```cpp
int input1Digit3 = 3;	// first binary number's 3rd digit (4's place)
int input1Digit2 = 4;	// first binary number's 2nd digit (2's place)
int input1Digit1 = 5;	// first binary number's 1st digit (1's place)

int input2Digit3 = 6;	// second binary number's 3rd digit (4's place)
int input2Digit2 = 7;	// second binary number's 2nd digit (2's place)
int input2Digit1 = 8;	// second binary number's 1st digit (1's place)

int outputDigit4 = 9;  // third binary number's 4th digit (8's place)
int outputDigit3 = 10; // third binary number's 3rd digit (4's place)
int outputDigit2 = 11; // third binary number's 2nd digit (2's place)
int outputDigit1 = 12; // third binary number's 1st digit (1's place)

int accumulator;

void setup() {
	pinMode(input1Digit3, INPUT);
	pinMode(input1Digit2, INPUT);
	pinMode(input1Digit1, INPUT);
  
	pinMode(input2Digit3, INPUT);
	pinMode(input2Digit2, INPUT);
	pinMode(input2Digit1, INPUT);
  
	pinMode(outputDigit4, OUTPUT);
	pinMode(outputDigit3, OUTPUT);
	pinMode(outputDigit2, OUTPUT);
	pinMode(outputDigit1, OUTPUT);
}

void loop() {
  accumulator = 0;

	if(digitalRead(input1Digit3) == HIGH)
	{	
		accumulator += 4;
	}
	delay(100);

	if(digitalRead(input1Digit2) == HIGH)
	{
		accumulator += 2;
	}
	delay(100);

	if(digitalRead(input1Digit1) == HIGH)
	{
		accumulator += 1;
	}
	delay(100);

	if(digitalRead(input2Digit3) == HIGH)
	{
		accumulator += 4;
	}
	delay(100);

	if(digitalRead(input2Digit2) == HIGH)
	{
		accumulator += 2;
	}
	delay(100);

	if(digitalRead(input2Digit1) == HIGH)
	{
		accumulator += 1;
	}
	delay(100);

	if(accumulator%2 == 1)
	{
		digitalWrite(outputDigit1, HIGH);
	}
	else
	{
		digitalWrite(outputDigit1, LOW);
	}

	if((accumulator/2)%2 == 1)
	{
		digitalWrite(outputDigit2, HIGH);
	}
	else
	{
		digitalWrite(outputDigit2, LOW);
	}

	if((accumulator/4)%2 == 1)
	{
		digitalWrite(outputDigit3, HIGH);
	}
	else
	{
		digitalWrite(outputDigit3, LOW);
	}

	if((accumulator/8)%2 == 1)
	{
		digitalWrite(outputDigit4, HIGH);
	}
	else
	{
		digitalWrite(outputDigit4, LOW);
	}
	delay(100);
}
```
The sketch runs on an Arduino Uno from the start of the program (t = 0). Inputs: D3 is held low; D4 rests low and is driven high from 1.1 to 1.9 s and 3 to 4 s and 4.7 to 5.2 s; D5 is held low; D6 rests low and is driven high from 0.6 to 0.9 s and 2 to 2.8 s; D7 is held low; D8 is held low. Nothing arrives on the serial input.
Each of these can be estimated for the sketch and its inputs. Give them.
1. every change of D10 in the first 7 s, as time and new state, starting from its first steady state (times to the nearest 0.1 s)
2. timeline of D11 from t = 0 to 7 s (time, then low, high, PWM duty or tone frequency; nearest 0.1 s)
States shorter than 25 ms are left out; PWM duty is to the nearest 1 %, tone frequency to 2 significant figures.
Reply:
0 s low; 2.7 s high; 3.4 s low
0 s low; 2 s high; 2.7 s low; 4.1 s high; 4.8 s low; 5.5 s high; 6.2 s low
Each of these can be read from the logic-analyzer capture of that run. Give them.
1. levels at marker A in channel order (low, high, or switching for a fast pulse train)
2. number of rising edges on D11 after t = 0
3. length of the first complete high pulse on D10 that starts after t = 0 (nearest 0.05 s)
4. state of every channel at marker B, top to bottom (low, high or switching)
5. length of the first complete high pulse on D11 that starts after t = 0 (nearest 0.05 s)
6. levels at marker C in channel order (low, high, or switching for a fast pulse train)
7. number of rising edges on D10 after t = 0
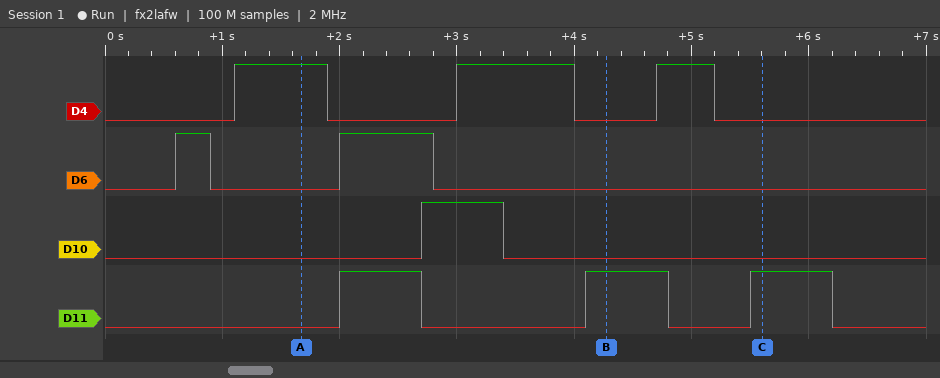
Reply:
D4 high, D6 low, D10 low, D11 low
3
0.70 s
D4 low, D6 low, D10 low, D11 high
0.70 s
D4 low, D6 low, D10 low, D11 high
1
